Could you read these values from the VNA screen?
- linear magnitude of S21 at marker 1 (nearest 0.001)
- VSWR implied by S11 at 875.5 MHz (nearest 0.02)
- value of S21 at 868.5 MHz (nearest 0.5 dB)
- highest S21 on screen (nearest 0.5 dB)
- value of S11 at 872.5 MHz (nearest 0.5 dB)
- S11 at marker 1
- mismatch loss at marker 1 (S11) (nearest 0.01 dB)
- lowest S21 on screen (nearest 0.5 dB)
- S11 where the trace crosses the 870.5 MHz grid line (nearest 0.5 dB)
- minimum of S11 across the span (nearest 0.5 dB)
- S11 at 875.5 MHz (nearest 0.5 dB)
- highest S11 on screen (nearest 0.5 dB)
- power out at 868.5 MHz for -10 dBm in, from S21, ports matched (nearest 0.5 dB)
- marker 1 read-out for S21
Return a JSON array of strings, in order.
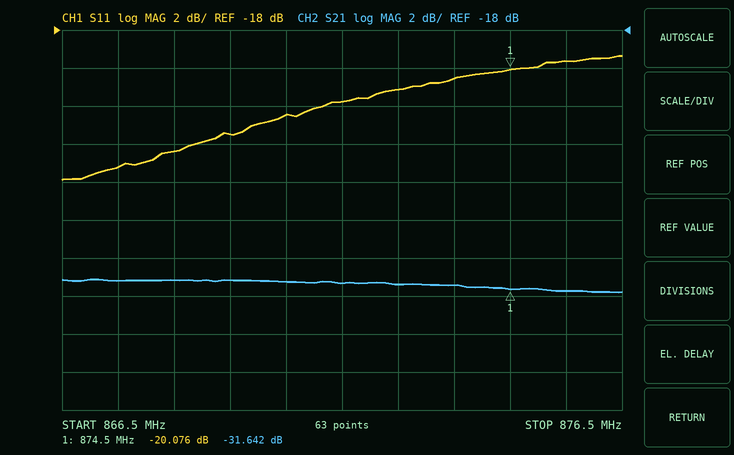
["0.026", "1.24", "-31.0 dB", "-31.0 dB", "-21.0 dB", "-20.076 dB", "0.04 dB", "-32.0 dB", "-22.5 dB", "-26.0 dB", "-19.5 dB", "-19.5 dB", "-41.0 dBm", "-31.642 dB"]
